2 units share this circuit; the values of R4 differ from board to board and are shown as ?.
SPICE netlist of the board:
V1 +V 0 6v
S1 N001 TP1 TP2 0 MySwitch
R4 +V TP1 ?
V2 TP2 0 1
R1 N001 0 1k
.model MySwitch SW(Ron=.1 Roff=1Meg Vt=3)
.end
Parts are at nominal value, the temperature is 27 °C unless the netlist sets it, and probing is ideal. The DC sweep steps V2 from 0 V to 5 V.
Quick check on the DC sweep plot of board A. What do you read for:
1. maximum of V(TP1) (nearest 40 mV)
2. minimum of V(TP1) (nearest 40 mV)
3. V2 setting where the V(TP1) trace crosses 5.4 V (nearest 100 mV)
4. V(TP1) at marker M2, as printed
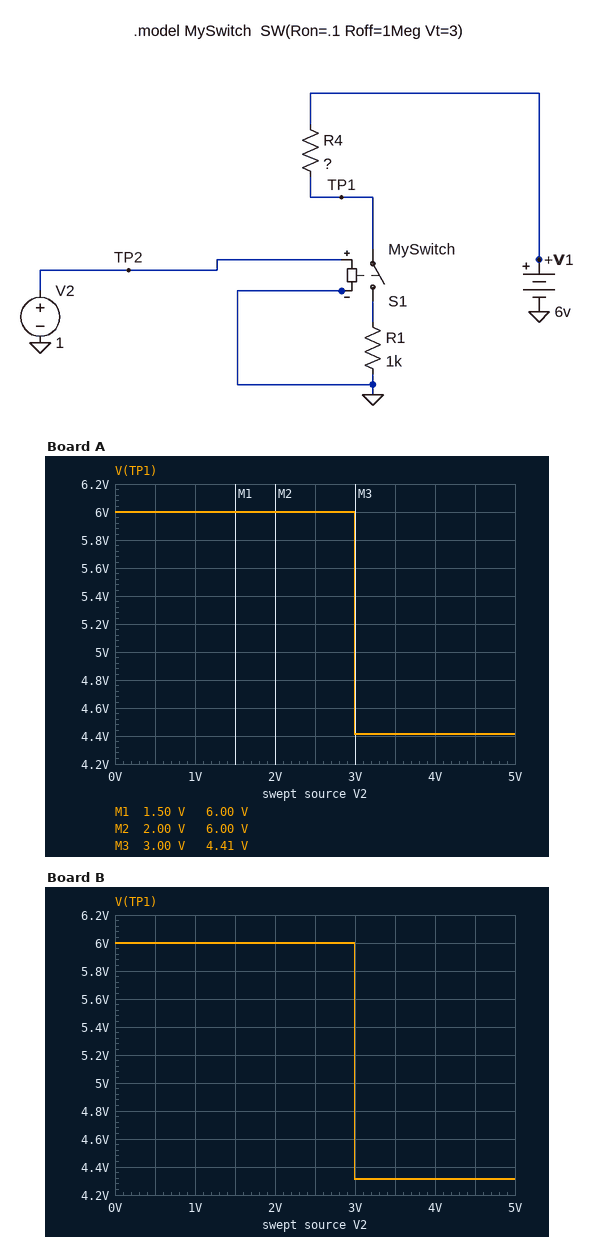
6.00 V
4.40 V
3.0 V
6.00 V
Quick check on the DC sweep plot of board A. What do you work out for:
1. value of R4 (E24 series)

360 Ω
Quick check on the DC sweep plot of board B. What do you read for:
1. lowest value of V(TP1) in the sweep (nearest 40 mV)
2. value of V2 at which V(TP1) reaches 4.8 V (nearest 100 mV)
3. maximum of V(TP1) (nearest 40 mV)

4.32 V
3.0 V
6.00 V
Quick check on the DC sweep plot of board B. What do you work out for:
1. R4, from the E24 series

390 Ω
